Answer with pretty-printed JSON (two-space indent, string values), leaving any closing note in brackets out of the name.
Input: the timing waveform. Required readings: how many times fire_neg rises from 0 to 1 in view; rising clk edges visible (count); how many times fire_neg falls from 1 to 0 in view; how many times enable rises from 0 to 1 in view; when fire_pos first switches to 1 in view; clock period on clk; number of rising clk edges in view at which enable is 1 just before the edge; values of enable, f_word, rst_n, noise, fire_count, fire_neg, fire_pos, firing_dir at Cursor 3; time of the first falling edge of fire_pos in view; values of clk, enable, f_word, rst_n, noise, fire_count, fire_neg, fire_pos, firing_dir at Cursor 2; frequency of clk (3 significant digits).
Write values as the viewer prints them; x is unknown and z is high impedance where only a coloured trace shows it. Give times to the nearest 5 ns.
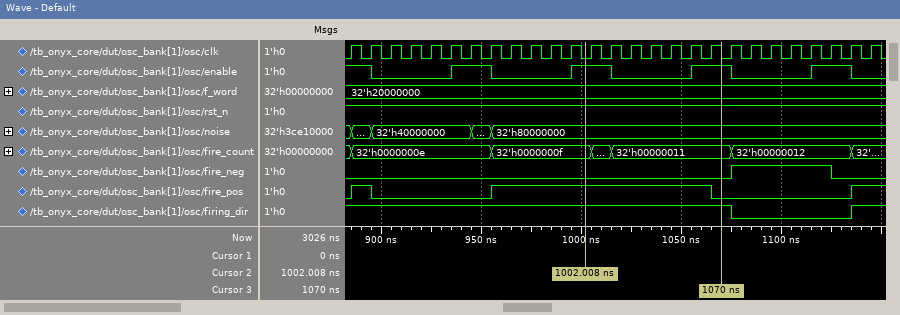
{
  "how many times fire_neg rises from 0 to 1 in view": "1",
  "rising clk edges visible": "27",
  "how many times fire_neg falls from 1 to 0 in view": "1",
  "how many times enable rises from 0 to 1 in view": "4",
  "when fire_pos first switches to 1 in view": "885 ns",
  "clock period on clk": "10 ns",
  "number of rising clk edges in view at which enable is 1 just before the edge": "10",
  "values of enable, f_word, rst_n, noise, fire_count, fire_neg, fire_pos, firing_dir at Cursor 3": "enable=1, f_word=32'h20000000, rst_n=1, noise=32'h80000000, fire_count=32'h00000011, fire_neg=0, fire_pos=0, firing_dir=1",
  "time of the first falling edge of fire_pos in view": "895 ns",
  "values of clk, enable, f_word, rst_n, noise, fire_count, fire_neg, fire_pos, firing_dir at Cursor 2": "clk=0, enable=1, f_word=32'h20000000, rst_n=1, noise=32'h80000000, fire_count=32'h0000000f, fire_neg=0, fire_pos=1, firing_dir=1",
  "frequency of clk": "100 MHz"
}
